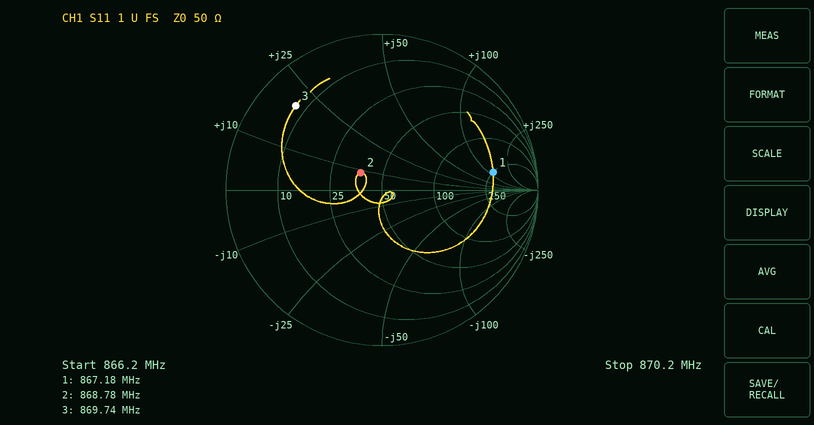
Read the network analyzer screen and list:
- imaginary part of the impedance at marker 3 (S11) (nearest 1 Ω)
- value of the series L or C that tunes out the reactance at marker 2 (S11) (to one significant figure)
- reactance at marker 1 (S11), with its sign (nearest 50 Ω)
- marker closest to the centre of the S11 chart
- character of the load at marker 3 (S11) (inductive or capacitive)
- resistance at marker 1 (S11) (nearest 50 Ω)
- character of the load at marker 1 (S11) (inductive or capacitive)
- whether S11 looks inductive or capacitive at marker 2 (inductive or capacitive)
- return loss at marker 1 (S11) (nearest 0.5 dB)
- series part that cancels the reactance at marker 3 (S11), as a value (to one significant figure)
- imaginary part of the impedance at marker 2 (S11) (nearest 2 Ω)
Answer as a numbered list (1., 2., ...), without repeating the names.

1. +20 Ω
2. 20 pF
3. +100 Ω
4. marker 2
5. inductive
6. 250 Ω
7. inductive
8. inductive
9. 3.0 dB
10. 9 pF
11. +8 Ω
